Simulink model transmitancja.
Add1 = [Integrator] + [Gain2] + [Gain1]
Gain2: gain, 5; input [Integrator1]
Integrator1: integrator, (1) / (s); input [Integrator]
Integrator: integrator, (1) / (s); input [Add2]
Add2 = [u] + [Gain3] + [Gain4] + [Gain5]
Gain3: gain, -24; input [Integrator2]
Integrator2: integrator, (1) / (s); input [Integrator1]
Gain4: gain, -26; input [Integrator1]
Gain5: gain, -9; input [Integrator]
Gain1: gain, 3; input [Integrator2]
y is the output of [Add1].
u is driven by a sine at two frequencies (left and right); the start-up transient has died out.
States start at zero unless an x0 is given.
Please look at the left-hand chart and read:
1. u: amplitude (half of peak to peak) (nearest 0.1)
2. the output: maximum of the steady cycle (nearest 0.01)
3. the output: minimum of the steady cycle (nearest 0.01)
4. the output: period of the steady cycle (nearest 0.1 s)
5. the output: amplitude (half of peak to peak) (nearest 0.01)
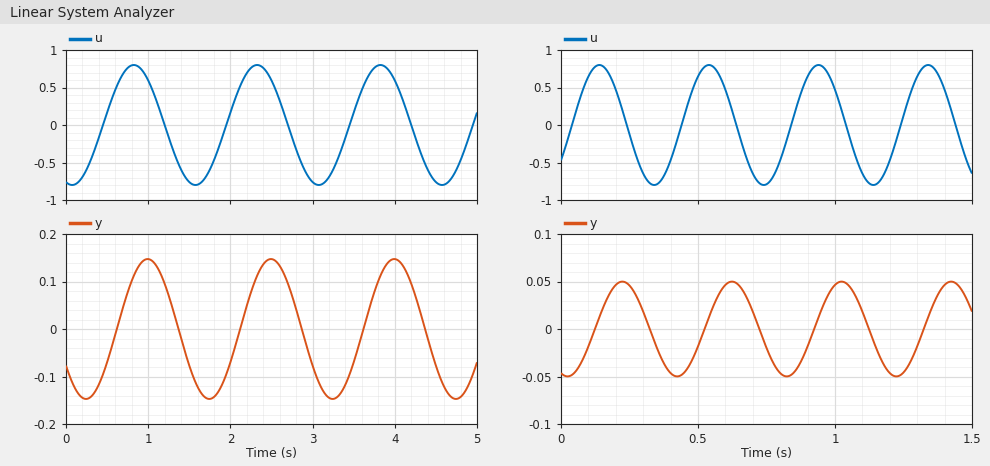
0.8
0.15
-0.15
1.5 s
0.15
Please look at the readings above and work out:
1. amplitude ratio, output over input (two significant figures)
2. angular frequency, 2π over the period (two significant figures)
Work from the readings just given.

0.19
4.2 rad/s
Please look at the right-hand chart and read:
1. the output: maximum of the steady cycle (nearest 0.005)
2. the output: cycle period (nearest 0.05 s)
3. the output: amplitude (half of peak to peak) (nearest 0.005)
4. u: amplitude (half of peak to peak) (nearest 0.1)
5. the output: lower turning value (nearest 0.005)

0.050
0.40 s
0.050
0.8
-0.050
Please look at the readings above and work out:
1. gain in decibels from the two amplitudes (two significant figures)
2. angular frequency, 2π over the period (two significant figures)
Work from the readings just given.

-24 dB
16 rad/s
